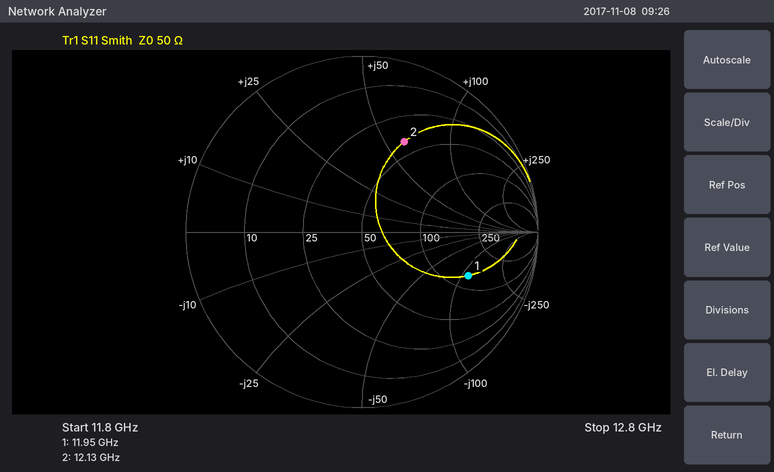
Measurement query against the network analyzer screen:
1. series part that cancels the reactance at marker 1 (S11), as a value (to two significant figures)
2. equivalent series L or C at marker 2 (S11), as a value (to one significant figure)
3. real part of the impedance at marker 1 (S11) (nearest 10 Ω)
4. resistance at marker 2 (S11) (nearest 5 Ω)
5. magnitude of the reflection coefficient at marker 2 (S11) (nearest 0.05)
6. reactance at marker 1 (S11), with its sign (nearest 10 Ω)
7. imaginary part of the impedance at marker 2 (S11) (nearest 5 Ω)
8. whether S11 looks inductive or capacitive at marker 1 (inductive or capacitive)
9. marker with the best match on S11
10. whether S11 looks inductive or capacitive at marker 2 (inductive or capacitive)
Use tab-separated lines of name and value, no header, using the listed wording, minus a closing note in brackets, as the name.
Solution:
series part that cancels the reactance at marker 1 (S11), as a value	1.5 nH
equivalent series L or C at marker 2 (S11), as a value	800 pH
real part of the impedance at marker 1 (S11)	130 Ω
resistance at marker 2 (S11)	40 Ω
magnitude of the reflection coefficient at marker 2 (S11)	0.55
reactance at marker 1 (S11), with its sign	-110 Ω
imaginary part of the impedance at marker 2 (S11)	+60 Ω
whether S11 looks inductive or capacitive at marker 1	capacitive
marker with the best match on S11	marker 2
whether S11 looks inductive or capacitive at marker 2	inductive
